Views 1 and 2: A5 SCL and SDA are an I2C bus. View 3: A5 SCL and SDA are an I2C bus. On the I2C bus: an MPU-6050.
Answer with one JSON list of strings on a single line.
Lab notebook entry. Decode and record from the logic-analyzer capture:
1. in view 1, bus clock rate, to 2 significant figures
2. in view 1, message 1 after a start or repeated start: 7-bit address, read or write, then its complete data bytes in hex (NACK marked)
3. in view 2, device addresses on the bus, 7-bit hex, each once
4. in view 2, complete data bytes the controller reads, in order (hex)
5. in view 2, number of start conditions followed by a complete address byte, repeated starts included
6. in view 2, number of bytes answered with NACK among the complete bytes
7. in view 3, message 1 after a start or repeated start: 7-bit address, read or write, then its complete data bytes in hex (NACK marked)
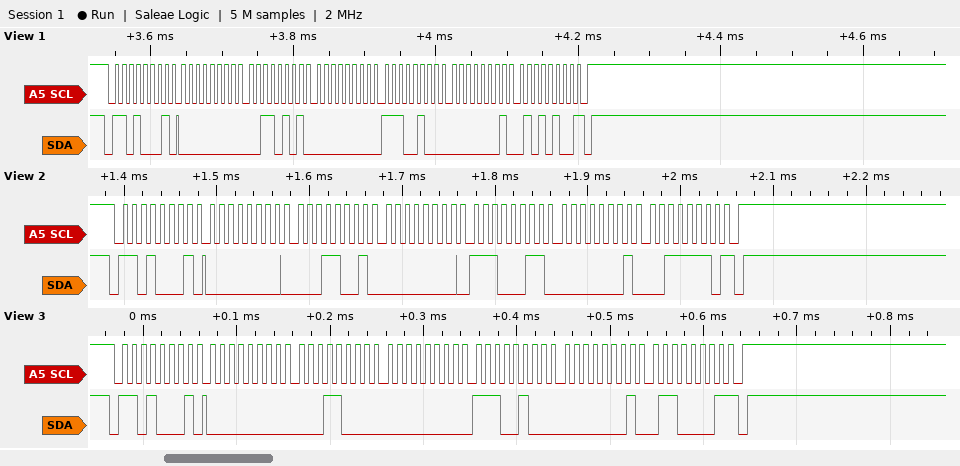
["100 kHz", "0x68 read: 00 35 00 E4 01 54 NACK", "0x68", "00 19 00 E3 01 3E", "1", "1", "0x68 read: 00 18 00 E4 01 61 NACK"]
